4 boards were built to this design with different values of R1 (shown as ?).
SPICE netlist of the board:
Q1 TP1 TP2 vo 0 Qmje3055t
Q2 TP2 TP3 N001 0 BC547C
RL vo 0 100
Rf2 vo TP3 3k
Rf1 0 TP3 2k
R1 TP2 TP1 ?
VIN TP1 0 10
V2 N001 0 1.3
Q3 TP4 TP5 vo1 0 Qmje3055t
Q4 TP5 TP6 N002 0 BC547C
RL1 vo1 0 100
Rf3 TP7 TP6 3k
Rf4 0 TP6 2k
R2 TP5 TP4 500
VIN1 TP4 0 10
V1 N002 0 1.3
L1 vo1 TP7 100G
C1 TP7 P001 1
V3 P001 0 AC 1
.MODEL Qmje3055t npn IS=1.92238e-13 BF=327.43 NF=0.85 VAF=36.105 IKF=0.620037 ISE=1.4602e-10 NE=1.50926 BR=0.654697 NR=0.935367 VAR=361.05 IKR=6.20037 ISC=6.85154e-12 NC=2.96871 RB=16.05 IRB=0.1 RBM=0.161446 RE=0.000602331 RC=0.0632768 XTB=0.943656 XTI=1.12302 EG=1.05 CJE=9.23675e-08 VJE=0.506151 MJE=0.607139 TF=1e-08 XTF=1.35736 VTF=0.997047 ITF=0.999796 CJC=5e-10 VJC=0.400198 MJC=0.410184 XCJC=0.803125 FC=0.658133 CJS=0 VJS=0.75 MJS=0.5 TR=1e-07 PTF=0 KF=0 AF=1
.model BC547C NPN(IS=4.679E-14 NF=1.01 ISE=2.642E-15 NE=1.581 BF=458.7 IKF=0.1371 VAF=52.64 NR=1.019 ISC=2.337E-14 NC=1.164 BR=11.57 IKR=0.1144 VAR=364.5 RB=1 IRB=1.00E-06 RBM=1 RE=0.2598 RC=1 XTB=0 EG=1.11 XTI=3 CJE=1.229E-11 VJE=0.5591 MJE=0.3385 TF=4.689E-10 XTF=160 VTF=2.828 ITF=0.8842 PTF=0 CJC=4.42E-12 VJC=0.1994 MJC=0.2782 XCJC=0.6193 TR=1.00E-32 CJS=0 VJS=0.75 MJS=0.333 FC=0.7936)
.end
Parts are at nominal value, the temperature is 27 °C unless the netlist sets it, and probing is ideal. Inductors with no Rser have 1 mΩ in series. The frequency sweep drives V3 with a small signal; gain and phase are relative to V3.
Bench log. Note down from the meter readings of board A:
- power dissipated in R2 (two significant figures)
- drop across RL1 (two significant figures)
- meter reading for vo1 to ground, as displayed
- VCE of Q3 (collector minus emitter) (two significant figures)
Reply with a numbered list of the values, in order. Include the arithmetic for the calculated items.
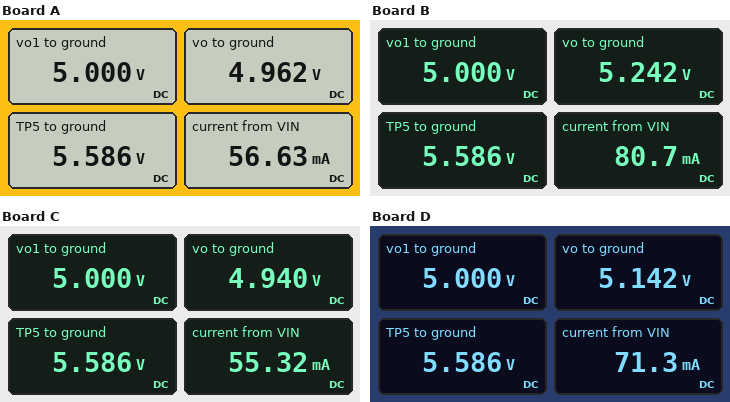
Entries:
1. (10 V - 5.586 V)^2 / 500 Ω = 39 mW
2. 5 V = 5.0 V
3. 5.000 V
4. 10 V - 5 V = 5.0 V
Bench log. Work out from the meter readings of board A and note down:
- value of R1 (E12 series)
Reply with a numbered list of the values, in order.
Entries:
1. 680 Ω
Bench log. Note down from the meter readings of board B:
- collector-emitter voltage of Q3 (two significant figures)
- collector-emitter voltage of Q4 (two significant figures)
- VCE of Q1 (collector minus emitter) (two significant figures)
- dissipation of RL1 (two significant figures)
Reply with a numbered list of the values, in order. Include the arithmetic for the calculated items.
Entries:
1. 10 V - 5 V = 5.0 V
2. 5.586 V - 1.3 V = 4.3 V
3. 10 V - 5.242 V = 4.8 V
4. (5 V)^2 / 100 Ω = 250 mW
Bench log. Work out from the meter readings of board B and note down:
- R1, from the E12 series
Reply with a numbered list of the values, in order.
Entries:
1. 150 Ω
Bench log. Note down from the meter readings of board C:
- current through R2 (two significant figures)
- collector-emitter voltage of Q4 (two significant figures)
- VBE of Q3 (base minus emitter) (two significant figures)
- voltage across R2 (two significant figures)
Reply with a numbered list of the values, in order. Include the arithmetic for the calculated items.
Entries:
1. (10 V - 5.586 V) / 500 Ω = 8.8 mA
2. 5.586 V - 1.3 V = 4.3 V
3. 5.586 V - 5 V = 590 mV
4. 10 V - 5.586 V = 4.4 V
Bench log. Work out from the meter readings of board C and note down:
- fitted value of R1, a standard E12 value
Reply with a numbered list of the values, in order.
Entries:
1. 820 Ω
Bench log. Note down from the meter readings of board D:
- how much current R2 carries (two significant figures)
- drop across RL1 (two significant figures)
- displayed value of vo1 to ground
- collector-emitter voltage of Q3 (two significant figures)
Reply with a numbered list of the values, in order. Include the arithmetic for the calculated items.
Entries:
1. (10 V - 5.586 V) / 500 Ω = 8.8 mA
2. 5 V = 5.0 V
3. 5.000 V
4. 10 V - 5 V = 5.0 V
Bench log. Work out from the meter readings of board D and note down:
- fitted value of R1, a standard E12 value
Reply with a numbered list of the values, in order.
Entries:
1. 220 Ω
